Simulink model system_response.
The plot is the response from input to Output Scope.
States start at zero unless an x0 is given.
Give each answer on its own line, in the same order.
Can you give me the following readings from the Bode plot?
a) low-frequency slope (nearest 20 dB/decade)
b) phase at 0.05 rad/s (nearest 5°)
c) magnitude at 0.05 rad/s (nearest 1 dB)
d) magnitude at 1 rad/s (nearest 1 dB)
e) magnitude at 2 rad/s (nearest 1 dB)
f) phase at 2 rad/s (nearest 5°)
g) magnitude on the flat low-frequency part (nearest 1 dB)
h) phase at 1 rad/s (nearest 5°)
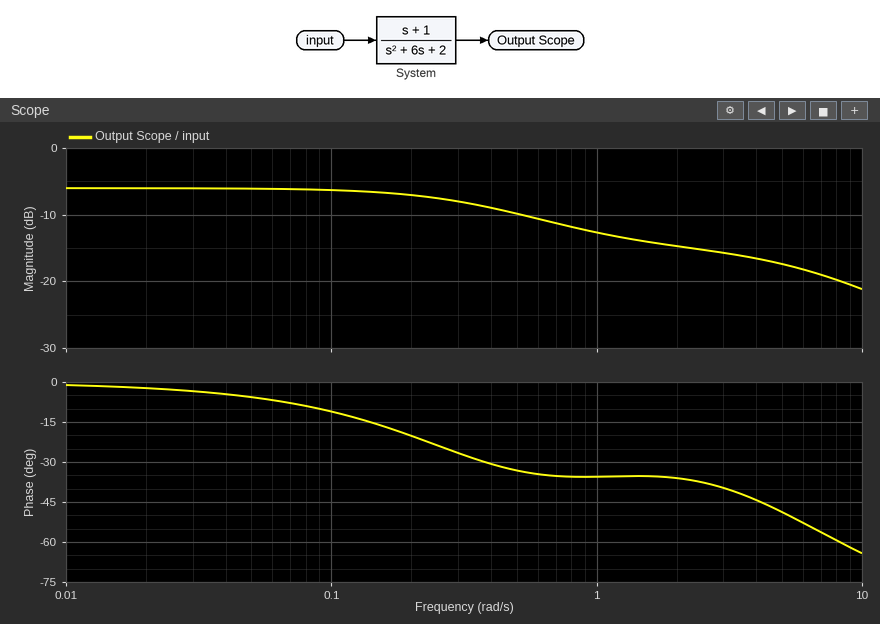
0 dB/decade
-5°
-6 dB
-13 dB
-15 dB
-35°
-6 dB
-35°
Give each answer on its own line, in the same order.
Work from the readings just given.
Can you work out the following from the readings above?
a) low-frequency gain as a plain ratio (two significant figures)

0.50
